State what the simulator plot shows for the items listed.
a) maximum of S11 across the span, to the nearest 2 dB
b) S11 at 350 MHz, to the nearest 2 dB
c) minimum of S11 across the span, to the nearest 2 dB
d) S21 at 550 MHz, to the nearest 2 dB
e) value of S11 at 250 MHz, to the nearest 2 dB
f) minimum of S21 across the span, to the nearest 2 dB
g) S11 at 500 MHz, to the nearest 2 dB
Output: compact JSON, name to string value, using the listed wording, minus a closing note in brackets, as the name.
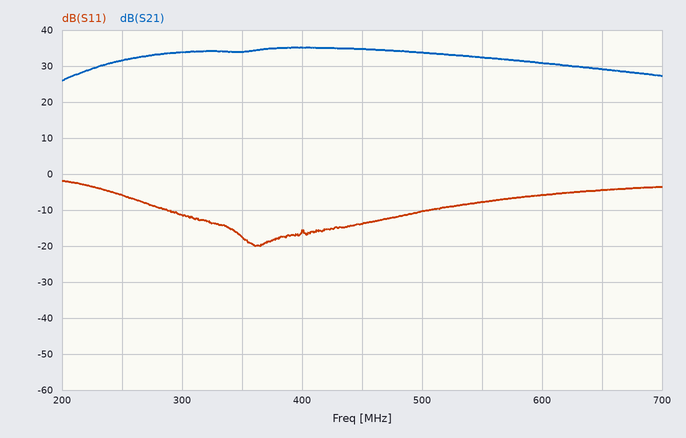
{"maximum of S11 across the span, to the nearest 2 dB": "-2 dB", "S11 at 350 MHz, to the nearest 2 dB": "-18 dB", "minimum of S11 across the span, to the nearest 2 dB": "-20 dB", "S21 at 550 MHz, to the nearest 2 dB": "32 dB", "value of S11 at 250 MHz, to the nearest 2 dB": "-6 dB", "minimum of S21 across the span, to the nearest 2 dB": "26 dB", "S11 at 500 MHz, to the nearest 2 dB": "-10 dB"}
